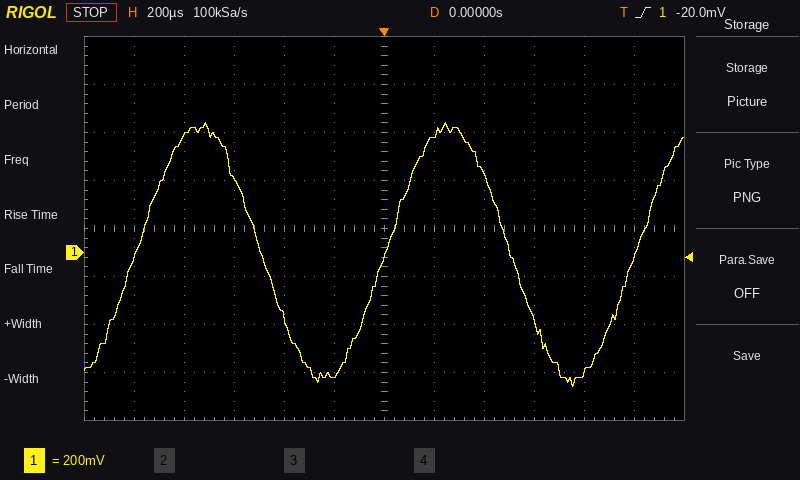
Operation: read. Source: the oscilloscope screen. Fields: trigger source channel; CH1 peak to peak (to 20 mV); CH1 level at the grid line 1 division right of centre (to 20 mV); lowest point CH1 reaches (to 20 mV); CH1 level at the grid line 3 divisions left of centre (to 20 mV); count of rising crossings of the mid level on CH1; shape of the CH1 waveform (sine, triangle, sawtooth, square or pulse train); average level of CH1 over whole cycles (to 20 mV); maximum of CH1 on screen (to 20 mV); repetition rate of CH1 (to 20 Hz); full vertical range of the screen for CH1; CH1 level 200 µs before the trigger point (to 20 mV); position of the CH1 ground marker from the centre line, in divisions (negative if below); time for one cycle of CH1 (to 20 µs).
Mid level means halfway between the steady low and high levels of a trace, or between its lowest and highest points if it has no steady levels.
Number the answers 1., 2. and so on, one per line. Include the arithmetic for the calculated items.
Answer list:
1. CH1
2. 540 mV − (-560 mV) = 1.10 V
3. 500 mV
4. -560 mV
5. 300 mV
6. 3
7. sine
8. (540 mV + (-560 mV)) / 2 ≈ 0 mV
9. 540 mV
10. 1 / 1.00 ms ≈ 1.00 kHz
11. 1.6 V
12. -520 mV
13. -0.5 div
14. 1.00 ms
